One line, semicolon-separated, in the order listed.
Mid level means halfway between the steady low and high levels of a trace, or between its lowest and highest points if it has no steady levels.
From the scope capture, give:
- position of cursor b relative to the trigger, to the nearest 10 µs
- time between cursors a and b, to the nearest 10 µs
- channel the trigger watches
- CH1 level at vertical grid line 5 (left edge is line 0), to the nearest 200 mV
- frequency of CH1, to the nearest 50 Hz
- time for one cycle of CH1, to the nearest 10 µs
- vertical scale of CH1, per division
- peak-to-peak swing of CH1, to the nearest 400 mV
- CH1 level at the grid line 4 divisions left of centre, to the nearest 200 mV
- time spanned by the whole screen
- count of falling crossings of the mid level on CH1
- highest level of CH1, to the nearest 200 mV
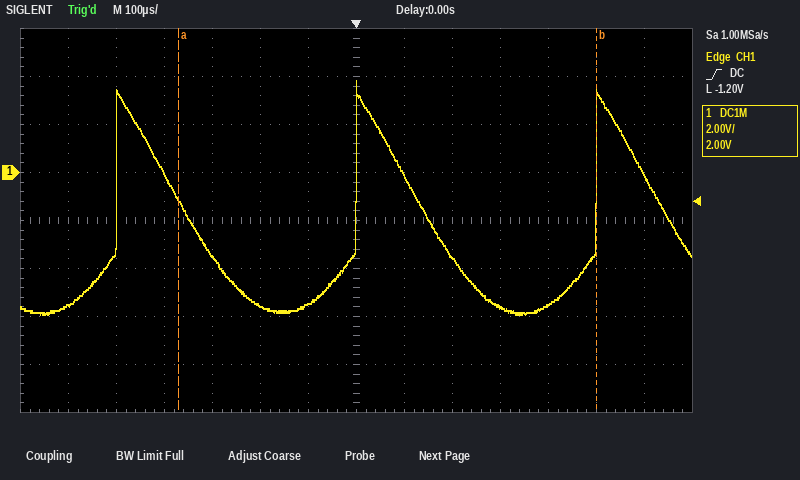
+500 µs; 870 µs; CH1; -5.6 V; 2.00 kHz; 500 µs; 2 V; 9.6 V; 0.0 V; 1.4 ms; 3; 3.8 V
